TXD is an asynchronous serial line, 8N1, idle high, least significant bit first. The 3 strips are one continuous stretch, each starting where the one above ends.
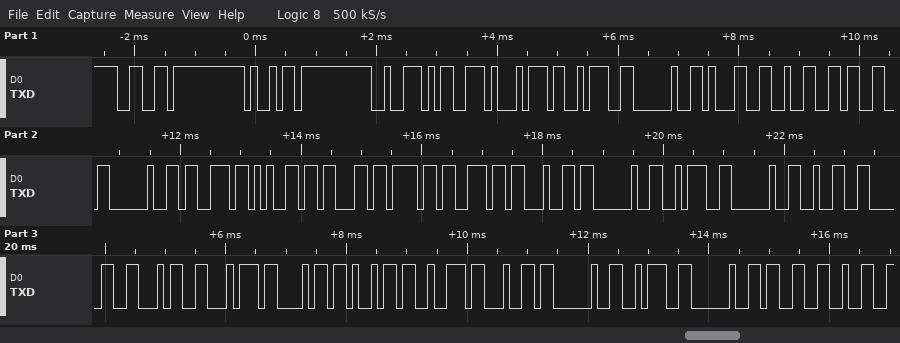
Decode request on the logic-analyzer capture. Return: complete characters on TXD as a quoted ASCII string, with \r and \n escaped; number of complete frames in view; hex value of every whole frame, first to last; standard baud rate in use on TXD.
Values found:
"first: 123 second : 204third : 32"
33
66 69 72 73 74 3A 20 31 32 33 20 73 65 63 6F 6E 64 20 3A 20 32 30 34 74 68 69 72 64 20 3A 20 33 32
9600 baud
